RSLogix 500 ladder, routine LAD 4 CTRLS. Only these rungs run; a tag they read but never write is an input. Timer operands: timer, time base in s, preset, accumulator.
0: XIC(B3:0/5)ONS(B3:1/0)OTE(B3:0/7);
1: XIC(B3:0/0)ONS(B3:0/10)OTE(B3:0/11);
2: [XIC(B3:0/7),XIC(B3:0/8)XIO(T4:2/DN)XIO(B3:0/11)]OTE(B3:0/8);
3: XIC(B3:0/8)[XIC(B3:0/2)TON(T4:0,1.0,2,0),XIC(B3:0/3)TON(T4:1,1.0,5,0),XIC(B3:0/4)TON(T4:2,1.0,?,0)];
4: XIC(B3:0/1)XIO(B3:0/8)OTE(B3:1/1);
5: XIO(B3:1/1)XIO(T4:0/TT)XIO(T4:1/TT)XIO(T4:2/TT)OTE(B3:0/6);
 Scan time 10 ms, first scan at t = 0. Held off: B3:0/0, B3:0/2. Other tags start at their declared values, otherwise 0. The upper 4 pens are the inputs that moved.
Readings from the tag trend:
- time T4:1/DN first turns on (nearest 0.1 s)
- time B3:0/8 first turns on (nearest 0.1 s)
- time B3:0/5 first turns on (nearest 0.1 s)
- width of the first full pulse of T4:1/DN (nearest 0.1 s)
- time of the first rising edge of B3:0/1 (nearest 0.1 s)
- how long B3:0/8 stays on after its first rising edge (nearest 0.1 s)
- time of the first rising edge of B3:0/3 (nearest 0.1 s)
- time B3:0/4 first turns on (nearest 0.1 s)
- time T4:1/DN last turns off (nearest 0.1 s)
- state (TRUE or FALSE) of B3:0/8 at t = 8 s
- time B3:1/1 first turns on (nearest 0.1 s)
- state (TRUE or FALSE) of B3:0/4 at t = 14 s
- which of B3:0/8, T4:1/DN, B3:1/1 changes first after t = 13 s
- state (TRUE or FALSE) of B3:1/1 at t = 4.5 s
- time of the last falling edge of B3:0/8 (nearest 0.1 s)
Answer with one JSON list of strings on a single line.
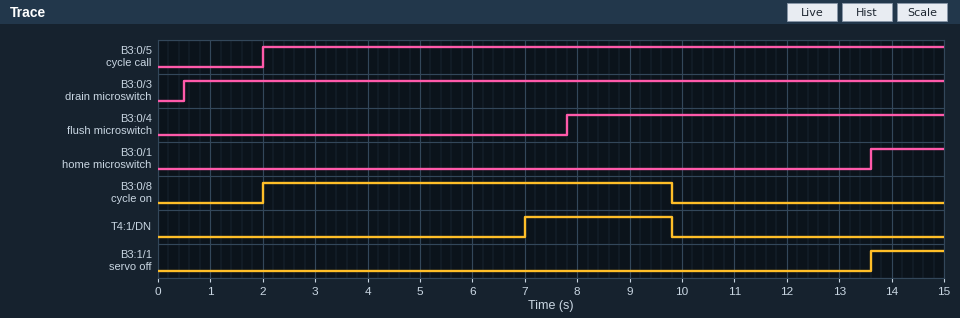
["7.0 s", "2.0 s", "2.0 s", "2.8 s", "13.6 s", "7.8 s", "0.5 s", "7.8 s", "9.8 s", "TRUE", "13.6 s", "TRUE", "B3:1/1", "FALSE", "9.8 s"]
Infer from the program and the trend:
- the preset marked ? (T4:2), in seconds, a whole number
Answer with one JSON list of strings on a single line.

["2 s"]
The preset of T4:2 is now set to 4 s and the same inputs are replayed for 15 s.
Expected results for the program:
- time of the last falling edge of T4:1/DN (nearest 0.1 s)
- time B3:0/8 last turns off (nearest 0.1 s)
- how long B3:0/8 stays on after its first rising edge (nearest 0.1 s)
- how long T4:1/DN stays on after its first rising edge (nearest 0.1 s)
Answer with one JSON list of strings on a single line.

["11.8 s", "11.8 s", "9.8 s", "4.8 s"]
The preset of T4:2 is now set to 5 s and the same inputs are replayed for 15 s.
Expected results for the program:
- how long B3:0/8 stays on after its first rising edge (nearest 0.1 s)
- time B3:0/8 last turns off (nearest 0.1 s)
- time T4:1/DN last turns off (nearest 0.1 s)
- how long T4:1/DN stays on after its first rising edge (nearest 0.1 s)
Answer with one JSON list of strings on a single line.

["10.8 s", "12.8 s", "12.8 s", "5.8 s"]
